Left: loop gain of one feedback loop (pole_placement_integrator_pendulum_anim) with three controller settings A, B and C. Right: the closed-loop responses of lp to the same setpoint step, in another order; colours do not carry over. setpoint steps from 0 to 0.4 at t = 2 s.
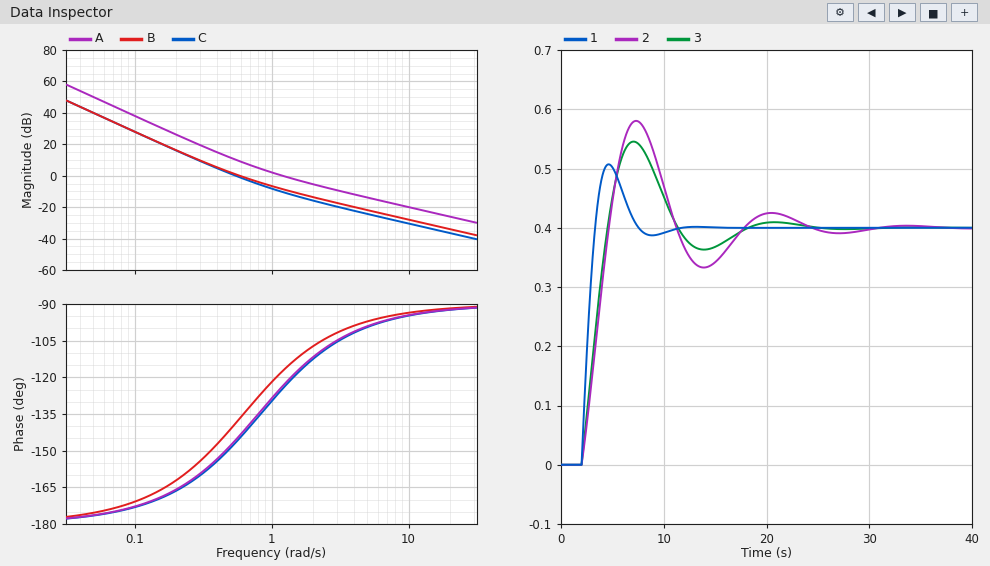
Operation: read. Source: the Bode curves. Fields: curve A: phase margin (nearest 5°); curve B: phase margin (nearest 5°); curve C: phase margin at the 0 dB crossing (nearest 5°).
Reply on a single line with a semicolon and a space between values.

55°; 45°; 35°
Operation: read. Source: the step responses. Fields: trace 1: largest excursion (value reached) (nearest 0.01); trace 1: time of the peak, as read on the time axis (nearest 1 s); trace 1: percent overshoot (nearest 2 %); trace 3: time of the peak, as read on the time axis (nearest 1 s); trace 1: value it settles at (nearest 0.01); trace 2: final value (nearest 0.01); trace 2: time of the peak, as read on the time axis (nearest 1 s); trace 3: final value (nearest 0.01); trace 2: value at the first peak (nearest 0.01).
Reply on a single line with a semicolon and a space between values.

0.51; 5 s; 26 %; 7 s; 0.40; 0.40; 7 s; 0.40; 0.58
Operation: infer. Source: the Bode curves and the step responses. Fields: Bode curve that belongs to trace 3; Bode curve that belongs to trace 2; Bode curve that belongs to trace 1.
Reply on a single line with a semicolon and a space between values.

B; C; A
